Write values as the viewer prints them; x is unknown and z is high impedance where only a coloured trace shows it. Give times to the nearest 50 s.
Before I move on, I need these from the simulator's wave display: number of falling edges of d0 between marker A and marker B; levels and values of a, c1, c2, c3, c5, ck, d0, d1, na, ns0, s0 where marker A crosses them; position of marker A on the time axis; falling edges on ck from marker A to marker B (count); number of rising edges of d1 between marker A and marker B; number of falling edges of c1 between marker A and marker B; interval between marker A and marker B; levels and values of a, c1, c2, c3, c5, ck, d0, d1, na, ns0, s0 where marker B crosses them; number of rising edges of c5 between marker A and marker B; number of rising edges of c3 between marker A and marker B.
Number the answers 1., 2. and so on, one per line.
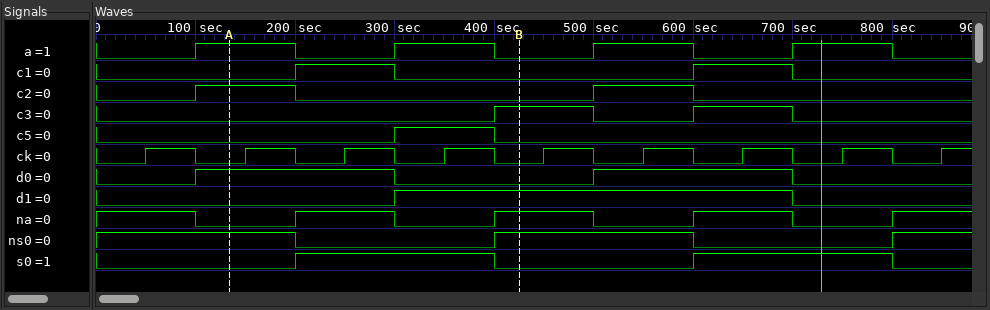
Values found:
1. 1
2. a=1, c1=0, c2=1, c3=0, c5=0, ck=0, d0=1, d1=0, na=0, ns0=1, s0=0
3. 150 s
4. 3
5. 1
6. 1
7. 300 s
8. a=0, c1=0, c2=0, c3=1, c5=0, ck=0, d0=0, d1=1, na=1, ns0=1, s0=0
9. 1
10. 1
